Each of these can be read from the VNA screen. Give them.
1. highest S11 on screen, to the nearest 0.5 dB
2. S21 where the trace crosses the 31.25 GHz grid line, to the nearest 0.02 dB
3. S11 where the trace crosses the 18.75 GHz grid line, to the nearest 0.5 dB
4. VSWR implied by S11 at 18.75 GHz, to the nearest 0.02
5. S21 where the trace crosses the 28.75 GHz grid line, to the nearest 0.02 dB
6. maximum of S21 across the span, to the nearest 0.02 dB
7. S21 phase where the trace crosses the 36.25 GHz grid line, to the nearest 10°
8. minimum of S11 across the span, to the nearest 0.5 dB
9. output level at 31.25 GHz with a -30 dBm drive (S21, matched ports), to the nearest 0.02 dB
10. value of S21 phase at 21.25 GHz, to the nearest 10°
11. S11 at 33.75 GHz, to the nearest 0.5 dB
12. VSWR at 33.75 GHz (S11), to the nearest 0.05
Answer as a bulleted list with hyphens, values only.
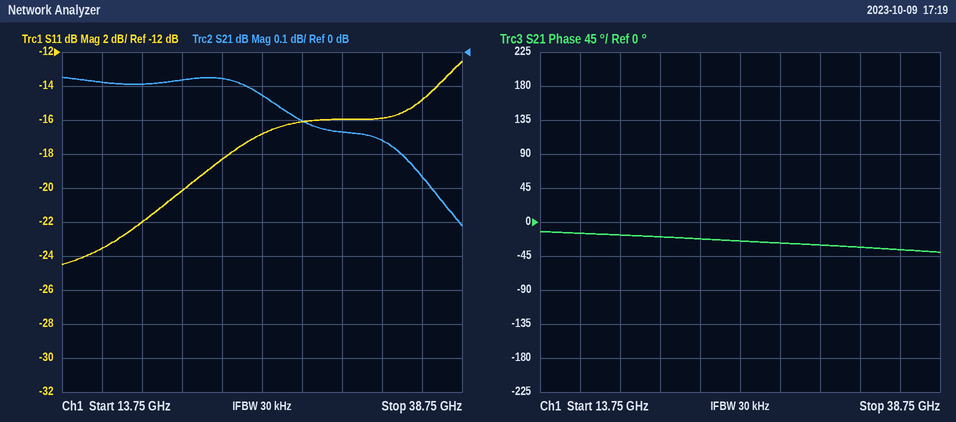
- -12.5 dB
- -0.24 dB
- -22.0 dB
- 1.18
- -0.20 dB
- -0.08 dB
- -40°
- -24.5 dB
- -30.24 dBm
- -20°
- -16.0 dB
- 1.40
